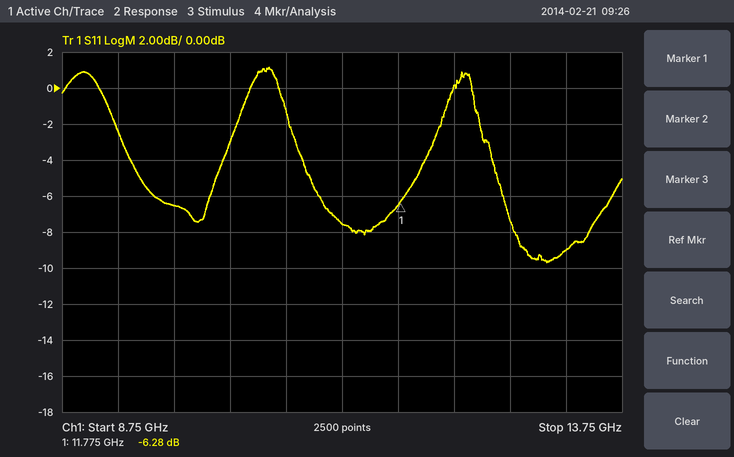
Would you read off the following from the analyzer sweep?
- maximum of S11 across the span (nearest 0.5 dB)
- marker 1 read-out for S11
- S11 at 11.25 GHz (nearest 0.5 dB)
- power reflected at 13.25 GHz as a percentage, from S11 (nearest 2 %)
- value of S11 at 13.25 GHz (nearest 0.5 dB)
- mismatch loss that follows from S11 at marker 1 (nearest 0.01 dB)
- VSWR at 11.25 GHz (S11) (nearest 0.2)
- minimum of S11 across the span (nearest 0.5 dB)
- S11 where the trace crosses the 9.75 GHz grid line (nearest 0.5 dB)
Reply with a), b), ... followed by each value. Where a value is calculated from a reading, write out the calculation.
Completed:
a) 1.0 dB
b) -6.28 dB
c) -7.5 dB
d) 10^(-9/10) ≈ 12.6 %, so 12 % to the nearest 2 %
e) -9.0 dB
f) −10 log10(1 − 10^(-6.28/10)) ≈ 1.17 dB
g) |Γ| = 10^(-7.5/20) = 0.4217; VSWR = (1 + 0.4217)/(1 − 0.4217) ≈ 2.46, so 2.4 to the nearest 0.2
h) -9.5 dB
i) -6.5 dB
